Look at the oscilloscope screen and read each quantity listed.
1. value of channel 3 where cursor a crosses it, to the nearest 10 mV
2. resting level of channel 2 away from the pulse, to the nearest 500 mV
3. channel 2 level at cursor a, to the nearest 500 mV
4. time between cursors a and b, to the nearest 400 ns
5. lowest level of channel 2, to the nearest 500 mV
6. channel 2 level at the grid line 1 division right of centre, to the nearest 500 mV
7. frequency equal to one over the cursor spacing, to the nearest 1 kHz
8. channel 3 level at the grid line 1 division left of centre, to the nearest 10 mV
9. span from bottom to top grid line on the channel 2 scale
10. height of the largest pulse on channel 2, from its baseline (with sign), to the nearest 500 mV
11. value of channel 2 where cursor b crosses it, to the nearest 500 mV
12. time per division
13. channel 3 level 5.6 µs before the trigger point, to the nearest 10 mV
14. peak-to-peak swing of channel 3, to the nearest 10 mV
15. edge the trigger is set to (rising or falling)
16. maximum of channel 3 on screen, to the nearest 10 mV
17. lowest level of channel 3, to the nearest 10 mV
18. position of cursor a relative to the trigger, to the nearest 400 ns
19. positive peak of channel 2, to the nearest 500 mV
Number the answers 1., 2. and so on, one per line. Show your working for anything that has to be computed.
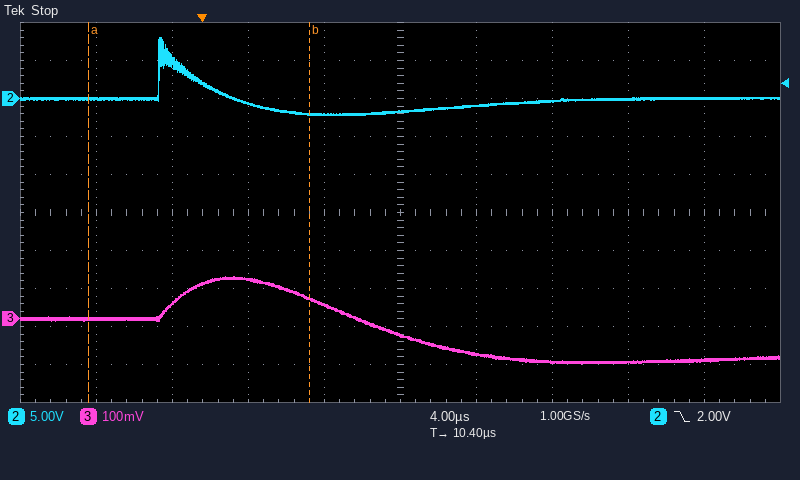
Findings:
1. 0 mV
2. 0.0 V
3. 0.0 V
4. 11.6 µs
5. -2.0 V
6. -1.0 V
7. 1 / 11.6 µs ≈ 86 kHz
8. 40 mV
9. 50 V
10. 8.0 V − (0.0 V) = +8.0 V
11. -2.0 V
12. 4 µs
13. 0 mV
14. 110 mV − (-120 mV) = 230 mV
15. falling
16. 110 mV
17. -120 mV
18. -6.0 µs
19. 8.0 V
